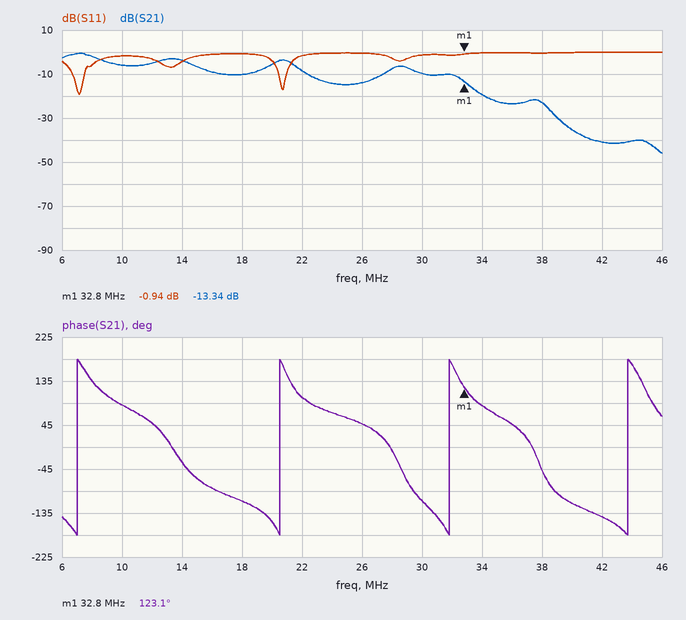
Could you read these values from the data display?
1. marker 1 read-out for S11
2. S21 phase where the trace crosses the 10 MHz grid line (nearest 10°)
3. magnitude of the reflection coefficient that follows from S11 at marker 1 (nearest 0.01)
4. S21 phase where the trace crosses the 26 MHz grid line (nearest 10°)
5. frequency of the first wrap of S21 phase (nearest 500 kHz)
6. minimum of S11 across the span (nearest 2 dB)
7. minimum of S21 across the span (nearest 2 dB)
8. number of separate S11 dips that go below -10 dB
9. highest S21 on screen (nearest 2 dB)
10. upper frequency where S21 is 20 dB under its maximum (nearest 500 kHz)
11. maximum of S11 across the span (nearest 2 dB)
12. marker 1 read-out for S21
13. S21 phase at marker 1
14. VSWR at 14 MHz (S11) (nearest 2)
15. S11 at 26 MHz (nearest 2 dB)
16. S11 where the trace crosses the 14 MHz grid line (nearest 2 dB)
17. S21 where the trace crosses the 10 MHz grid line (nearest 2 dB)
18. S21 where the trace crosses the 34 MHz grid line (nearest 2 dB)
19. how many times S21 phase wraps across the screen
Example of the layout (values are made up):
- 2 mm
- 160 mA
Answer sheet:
- -0.94 dB
- 90°
- 0.90
- 50°
- 7.0 MHz
- -20 dB
- -46 dB
- 2
- 0 dB
- 34.5 MHz
- 0 dB
- -13.34 dB
- 123.1°
- 4
- 0 dB
- -4 dB
- -6 dB
- -20 dB
- 4
